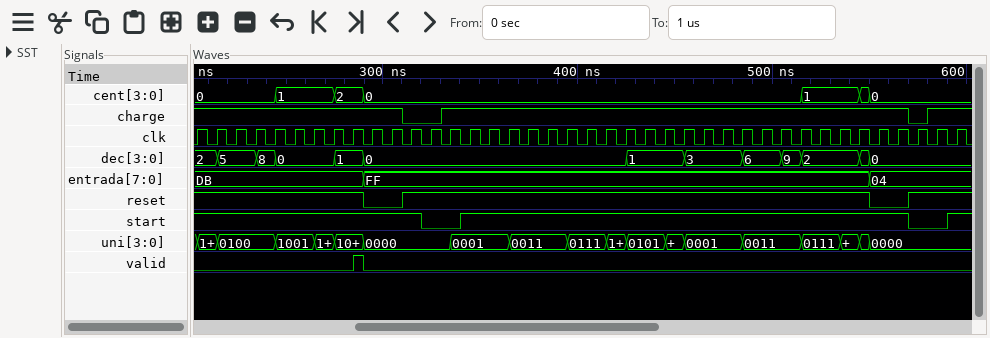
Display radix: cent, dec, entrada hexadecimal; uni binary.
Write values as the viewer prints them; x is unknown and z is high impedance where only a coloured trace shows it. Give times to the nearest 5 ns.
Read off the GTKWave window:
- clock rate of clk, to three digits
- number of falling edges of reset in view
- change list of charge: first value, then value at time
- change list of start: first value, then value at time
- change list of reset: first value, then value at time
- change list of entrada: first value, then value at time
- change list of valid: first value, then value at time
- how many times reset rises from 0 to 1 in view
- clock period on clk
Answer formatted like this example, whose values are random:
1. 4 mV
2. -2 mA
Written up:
1. 100 MHz
2. 2
3. 1, 0 at 310 ns, 1 at 330 ns, 0 at 570 ns, 1 at 580 ns
4. 1, 0 at 320 ns, 1 at 340 ns, 0 at 570 ns, 1 at 590 ns
5. 1, 0 at 290 ns, 1 at 310 ns, 0 at 550 ns, 1 at 570 ns
6. DB, FF at 290 ns, 04 at 550 ns
7. 0, 1 at 285 ns, 0 at 290 ns
8. 2
9. 10 ns
